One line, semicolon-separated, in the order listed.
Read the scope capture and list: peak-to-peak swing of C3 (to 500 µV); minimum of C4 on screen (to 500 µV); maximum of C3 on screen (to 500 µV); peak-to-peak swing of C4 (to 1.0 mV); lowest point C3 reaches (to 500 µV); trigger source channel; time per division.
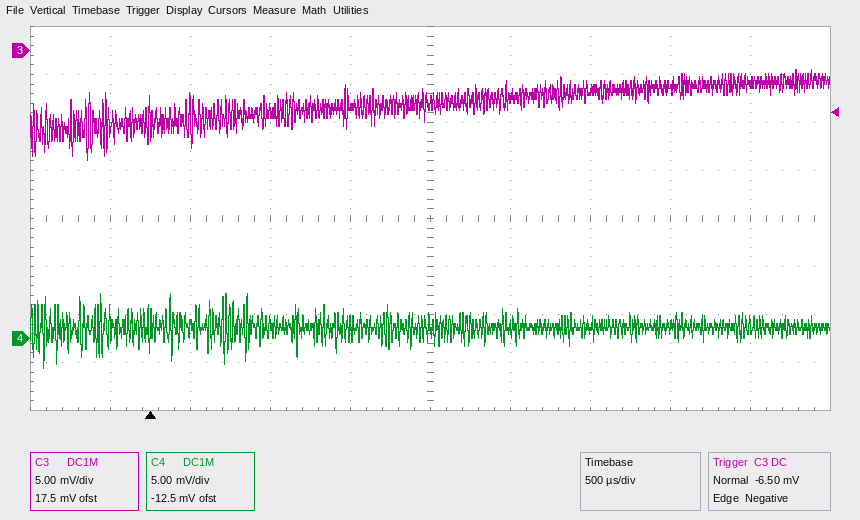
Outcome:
9.5 mV; -3.0 mV; -2.0 mV; 8.0 mV; -11.5 mV; C3; 500 µs
